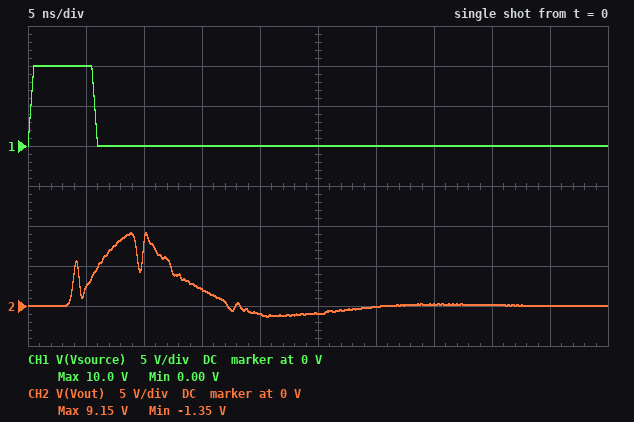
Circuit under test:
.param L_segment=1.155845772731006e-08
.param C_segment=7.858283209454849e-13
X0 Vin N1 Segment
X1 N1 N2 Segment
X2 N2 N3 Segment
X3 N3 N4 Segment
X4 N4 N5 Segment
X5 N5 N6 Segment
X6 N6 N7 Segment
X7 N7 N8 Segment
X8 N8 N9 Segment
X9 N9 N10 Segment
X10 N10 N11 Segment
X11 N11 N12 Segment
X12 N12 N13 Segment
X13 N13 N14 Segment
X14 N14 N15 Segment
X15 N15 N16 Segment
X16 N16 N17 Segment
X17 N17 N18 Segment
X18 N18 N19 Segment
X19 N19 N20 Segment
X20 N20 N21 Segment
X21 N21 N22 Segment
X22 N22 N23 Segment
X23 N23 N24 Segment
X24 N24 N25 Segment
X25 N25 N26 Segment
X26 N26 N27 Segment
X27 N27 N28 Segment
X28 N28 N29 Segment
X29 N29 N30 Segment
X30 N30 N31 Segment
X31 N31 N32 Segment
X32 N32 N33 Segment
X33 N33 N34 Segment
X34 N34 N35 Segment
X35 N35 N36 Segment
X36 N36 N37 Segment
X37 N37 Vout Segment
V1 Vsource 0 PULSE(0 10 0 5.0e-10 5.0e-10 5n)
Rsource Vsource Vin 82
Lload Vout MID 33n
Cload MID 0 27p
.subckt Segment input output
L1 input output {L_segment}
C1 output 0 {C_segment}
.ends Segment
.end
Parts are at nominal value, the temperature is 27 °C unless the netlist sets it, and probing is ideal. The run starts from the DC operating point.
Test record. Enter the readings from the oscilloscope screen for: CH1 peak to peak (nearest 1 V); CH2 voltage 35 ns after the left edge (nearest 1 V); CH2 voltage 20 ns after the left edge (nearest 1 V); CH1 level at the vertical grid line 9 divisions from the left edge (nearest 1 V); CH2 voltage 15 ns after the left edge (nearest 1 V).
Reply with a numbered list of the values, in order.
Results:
1. 10 V
2. 0 V
3. -1 V
4. 0 V
5. 2 V
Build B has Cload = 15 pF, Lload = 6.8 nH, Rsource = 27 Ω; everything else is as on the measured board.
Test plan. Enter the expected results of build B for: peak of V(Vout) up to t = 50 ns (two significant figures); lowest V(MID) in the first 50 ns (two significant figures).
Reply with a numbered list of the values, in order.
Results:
1. 15 V
2. -10 V
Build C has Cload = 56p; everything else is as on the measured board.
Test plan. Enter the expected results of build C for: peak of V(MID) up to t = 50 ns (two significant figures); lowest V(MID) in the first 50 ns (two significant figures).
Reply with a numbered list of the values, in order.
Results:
1. 6.6 V
2. -500 mV
